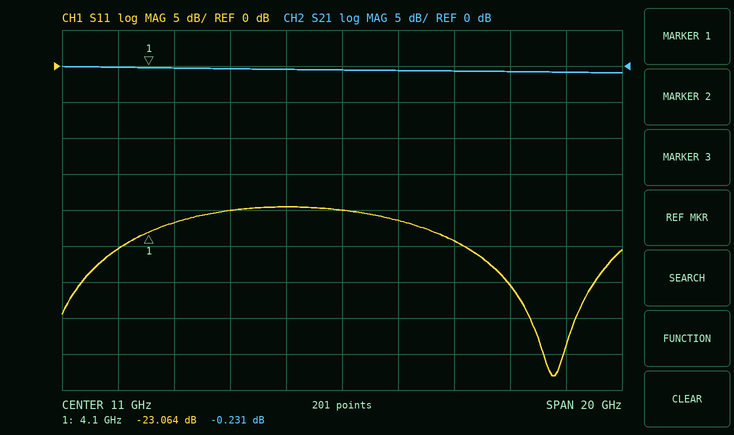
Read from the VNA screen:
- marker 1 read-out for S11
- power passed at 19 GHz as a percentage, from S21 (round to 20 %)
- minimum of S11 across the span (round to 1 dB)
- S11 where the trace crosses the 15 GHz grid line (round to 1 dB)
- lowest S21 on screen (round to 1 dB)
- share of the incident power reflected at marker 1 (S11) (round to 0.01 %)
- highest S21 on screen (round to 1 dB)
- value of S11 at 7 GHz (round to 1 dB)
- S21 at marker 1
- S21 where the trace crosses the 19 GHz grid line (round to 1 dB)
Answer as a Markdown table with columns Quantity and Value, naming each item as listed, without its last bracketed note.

| Quantity | Value |
|---|---|
| marker 1 read-out for S11 | -23.064 dB |
| power passed at 19 GHz as a percentage, from S21 | 80 % |
| minimum of S11 across the span | -43 dB |
| S11 where the trace crosses the 15 GHz grid line | -24 dB |
| lowest S21 on screen | -1 dB |
| share of the incident power reflected at marker 1 (S11) | 0.49 % |
| highest S21 on screen | 0 dB |
| value of S11 at 7 GHz | -20 dB |
| S21 at marker 1 | -0.231 dB |
| S21 where the trace crosses the 19 GHz grid line | -1 dB |
